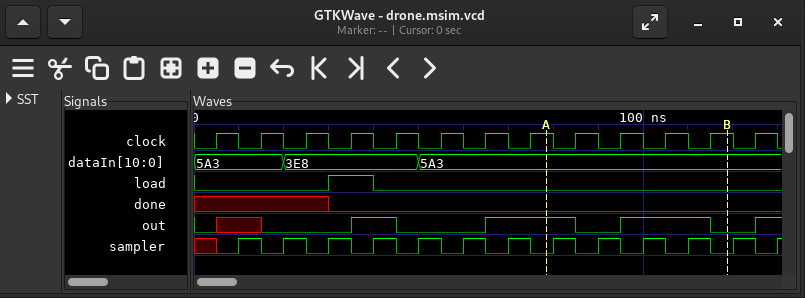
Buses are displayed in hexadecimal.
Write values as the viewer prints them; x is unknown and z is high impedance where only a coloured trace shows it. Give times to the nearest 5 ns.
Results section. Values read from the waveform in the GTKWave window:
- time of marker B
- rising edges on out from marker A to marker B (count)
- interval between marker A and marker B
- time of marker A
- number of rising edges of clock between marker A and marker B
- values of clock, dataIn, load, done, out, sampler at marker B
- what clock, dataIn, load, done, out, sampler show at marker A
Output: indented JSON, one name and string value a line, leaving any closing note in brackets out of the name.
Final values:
{
  "time of marker B": "120 ns",
  "rising edges on out from marker A to marker B": "1",
  "interval between marker A and marker B": "40 ns",
  "time of marker A": "80 ns",
  "number of rising edges of clock between marker A and marker B": "4",
  "values of clock, dataIn, load, done, out, sampler at marker B": "clock=1, dataIn=5A3, load=0, done=0, out=0, sampler=0",
  "what clock, dataIn, load, done, out, sampler show at marker A": "clock=1, dataIn=5A3, load=0, done=0, out=1, sampler=0"
}
